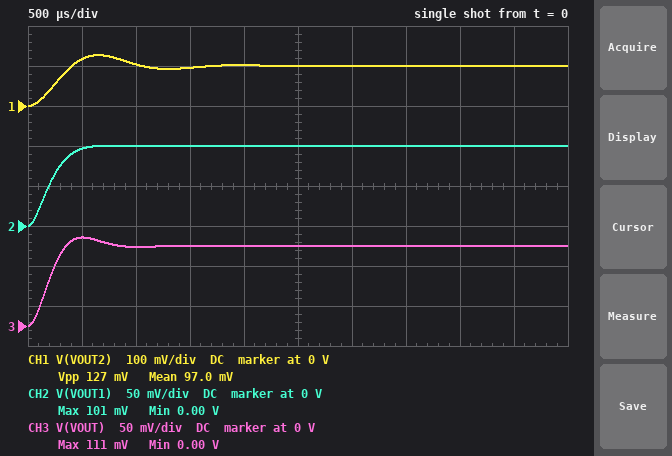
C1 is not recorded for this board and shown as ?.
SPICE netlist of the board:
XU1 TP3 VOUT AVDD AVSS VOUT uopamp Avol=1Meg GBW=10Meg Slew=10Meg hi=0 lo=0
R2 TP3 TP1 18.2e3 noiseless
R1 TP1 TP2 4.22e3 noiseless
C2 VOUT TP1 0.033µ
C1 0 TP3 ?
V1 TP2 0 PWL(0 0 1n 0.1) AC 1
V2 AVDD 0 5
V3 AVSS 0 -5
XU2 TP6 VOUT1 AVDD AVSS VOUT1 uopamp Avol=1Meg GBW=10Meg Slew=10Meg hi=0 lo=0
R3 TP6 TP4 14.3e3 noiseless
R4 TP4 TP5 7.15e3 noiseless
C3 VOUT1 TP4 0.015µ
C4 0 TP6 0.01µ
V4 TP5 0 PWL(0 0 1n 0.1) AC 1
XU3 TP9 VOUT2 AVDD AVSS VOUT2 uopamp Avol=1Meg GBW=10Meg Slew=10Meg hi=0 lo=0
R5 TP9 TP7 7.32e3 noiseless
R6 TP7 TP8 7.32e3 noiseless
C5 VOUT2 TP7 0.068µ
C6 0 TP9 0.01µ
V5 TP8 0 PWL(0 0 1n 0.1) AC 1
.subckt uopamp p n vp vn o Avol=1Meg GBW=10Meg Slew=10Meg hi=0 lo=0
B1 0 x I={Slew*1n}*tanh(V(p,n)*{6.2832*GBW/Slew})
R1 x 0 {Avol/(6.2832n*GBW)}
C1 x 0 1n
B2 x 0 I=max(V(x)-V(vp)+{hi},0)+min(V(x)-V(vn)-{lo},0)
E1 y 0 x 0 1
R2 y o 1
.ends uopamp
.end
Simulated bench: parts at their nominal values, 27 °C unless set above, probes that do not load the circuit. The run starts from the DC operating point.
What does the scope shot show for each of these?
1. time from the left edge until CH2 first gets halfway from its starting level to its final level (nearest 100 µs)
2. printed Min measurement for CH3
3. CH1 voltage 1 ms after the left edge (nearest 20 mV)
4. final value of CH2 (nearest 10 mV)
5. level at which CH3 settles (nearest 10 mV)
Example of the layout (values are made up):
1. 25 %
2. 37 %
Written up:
1. 200 µs
2. 0.00 V
3. 100 mV
4. 100 mV
5. 100 mV
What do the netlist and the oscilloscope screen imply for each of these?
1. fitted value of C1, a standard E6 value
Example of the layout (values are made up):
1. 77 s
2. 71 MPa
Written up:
1. 6.8 nF
